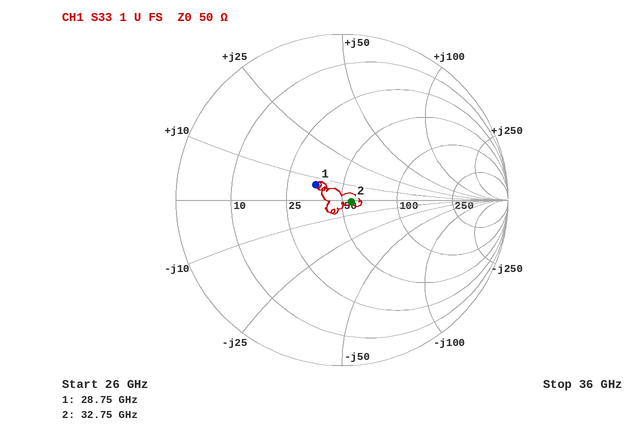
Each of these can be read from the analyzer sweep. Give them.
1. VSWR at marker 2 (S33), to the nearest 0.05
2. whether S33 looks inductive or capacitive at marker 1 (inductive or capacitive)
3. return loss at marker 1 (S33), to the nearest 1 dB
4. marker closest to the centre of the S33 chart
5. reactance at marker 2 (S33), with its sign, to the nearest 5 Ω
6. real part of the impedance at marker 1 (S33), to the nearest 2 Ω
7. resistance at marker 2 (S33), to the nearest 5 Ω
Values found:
1.10
inductive
15 dB
marker 2
0 Ω
36 Ω
55 Ω
